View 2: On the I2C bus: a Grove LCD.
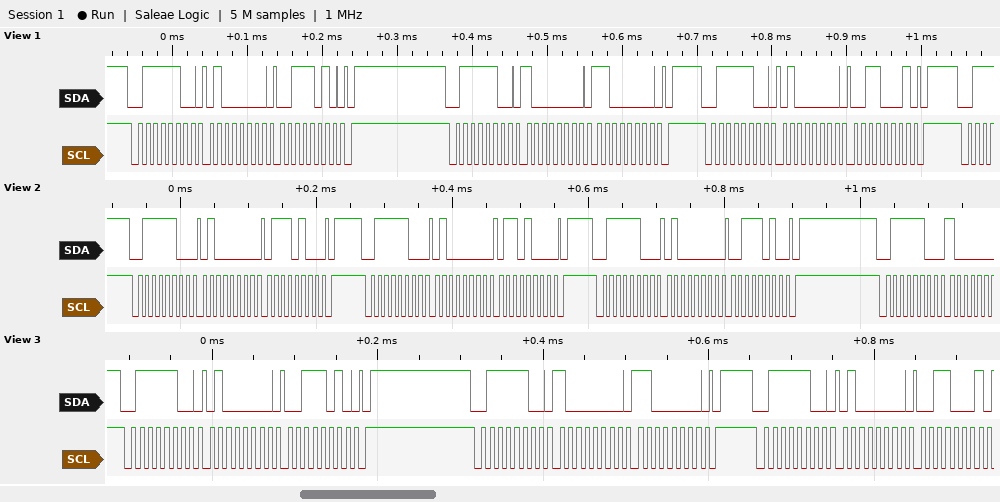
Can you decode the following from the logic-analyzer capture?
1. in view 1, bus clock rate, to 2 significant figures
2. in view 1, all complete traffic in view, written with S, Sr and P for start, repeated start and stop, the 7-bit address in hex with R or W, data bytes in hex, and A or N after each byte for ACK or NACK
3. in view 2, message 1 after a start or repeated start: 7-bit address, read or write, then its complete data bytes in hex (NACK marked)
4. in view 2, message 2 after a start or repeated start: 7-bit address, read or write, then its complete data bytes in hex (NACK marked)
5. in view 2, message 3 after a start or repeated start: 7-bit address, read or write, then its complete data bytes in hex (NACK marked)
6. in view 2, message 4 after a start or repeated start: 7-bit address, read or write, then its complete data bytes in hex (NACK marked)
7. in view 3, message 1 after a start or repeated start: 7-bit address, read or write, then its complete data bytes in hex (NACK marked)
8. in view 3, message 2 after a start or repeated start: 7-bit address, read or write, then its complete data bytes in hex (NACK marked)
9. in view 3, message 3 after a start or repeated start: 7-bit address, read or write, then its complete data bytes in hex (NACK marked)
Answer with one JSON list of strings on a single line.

["100 kHz", "S 3EW A 40 A 3A A P S 3EW A 80 A C0 A P S 3EW A 40 A 31 A P", "0x3E write: 40 74", "0x3E write: 40 68", "0x3E write: 40 3A", "0x3E write", "0x3E write: 40 3A", "0x3E write: 80 C0", "0x3E write: 40 31"]
